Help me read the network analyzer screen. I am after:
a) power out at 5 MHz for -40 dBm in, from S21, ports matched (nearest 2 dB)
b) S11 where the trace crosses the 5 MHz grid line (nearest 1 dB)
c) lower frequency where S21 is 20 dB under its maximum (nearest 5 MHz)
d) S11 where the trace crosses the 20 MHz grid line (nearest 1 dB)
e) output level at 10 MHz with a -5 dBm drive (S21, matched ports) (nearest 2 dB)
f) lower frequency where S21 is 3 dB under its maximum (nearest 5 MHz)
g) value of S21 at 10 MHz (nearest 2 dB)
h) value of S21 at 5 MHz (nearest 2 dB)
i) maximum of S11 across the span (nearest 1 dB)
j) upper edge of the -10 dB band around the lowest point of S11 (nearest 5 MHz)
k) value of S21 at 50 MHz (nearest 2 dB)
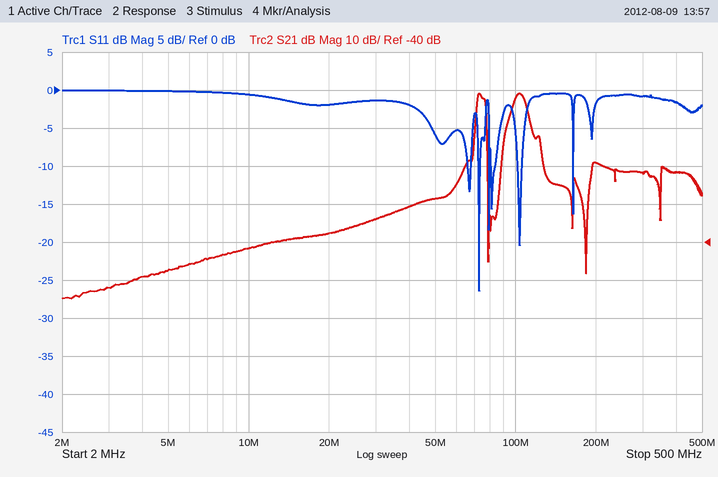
-88 dBm
0 dB
65 MHz
-2 dB
-46 dBm
70 MHz
-42 dB
-48 dB
0 dB
75 MHz
-28 dB
